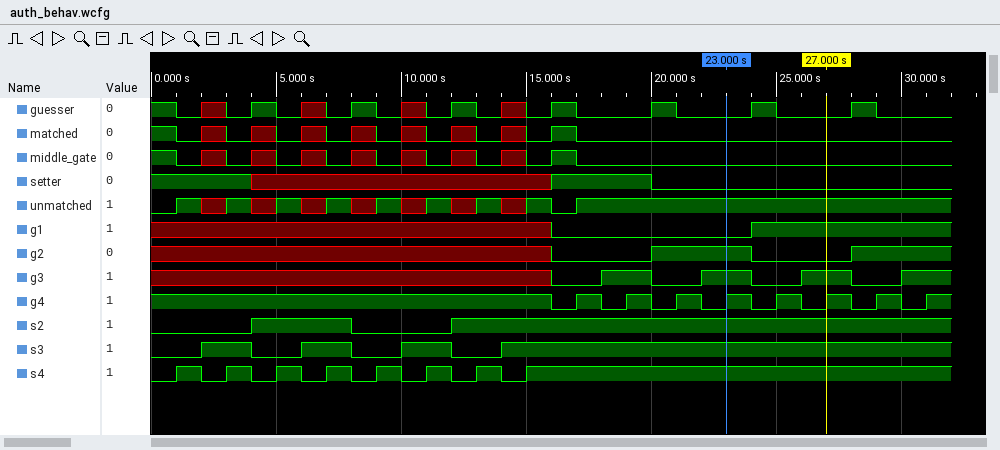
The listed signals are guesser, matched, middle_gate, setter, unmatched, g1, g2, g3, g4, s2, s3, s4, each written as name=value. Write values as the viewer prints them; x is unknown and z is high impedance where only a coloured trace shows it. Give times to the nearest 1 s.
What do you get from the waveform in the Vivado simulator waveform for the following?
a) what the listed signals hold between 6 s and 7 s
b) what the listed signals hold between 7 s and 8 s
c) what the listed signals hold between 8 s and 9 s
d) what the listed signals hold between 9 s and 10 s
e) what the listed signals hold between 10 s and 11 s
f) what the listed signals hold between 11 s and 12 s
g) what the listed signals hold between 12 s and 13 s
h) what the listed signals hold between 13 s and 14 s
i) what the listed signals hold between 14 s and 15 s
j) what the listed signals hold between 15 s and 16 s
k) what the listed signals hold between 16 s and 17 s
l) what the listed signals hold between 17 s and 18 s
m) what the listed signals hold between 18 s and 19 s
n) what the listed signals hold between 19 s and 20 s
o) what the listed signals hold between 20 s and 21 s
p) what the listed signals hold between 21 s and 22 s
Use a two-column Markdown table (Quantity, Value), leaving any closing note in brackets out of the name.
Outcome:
| Quantity | Value |
|---|---|
| what the listed signals hold between 6 s and 7 s | guesser=x, matched=x, middle_gate=x, setter=x, unmatched=x, g1=x, g2=x, g3=x, g4=1, s2=1, s3=1, s4=0 |
| what the listed signals hold between 7 s and 8 s | guesser=0, matched=0, middle_gate=0, setter=x, unmatched=1, g1=x, g2=x, g3=x, g4=1, s2=1, s3=1, s4=1 |
| what the listed signals hold between 8 s and 9 s | guesser=1, matched=x, middle_gate=x, setter=x, unmatched=x, g1=x, g2=x, g3=x, g4=1, s2=0, s3=0, s4=0 |
| what the listed signals hold between 9 s and 10 s | guesser=0, matched=0, middle_gate=0, setter=x, unmatched=1, g1=x, g2=x, g3=x, g4=1, s2=0, s3=0, s4=1 |
| what the listed signals hold between 10 s and 11 s | guesser=x, matched=x, middle_gate=x, setter=x, unmatched=x, g1=x, g2=x, g3=x, g4=1, s2=0, s3=1, s4=0 |
| what the listed signals hold between 11 s and 12 s | guesser=0, matched=0, middle_gate=0, setter=x, unmatched=1, g1=x, g2=x, g3=x, g4=1, s2=0, s3=1, s4=1 |
| what the listed signals hold between 12 s and 13 s | guesser=1, matched=x, middle_gate=x, setter=x, unmatched=x, g1=x, g2=x, g3=x, g4=1, s2=1, s3=0, s4=0 |
| what the listed signals hold between 13 s and 14 s | guesser=0, matched=0, middle_gate=0, setter=x, unmatched=1, g1=x, g2=x, g3=x, g4=1, s2=1, s3=0, s4=1 |
| what the listed signals hold between 14 s and 15 s | guesser=x, matched=x, middle_gate=x, setter=x, unmatched=x, g1=x, g2=x, g3=x, g4=1, s2=1, s3=1, s4=0 |
| what the listed signals hold between 15 s and 16 s | guesser=0, matched=0, middle_gate=0, setter=x, unmatched=1, g1=x, g2=x, g3=x, g4=1, s2=1, s3=1, s4=1 |
| what the listed signals hold between 16 s and 17 s | guesser=1, matched=1, middle_gate=1, setter=1, unmatched=0, g1=0, g2=0, g3=0, g4=0, s2=1, s3=1, s4=1 |
| what the listed signals hold between 17 s and 18 s | guesser=0, matched=0, middle_gate=0, setter=1, unmatched=1, g1=0, g2=0, g3=0, g4=1, s2=1, s3=1, s4=1 |
| what the listed signals hold between 18 s and 19 s | guesser=0, matched=0, middle_gate=0, setter=1, unmatched=1, g1=0, g2=0, g3=1, g4=0, s2=1, s3=1, s4=1 |
| what the listed signals hold between 19 s and 20 s | guesser=0, matched=0, middle_gate=0, setter=1, unmatched=1, g1=0, g2=0, g3=1, g4=1, s2=1, s3=1, s4=1 |
| what the listed signals hold between 20 s and 21 s | guesser=1, matched=0, middle_gate=0, setter=0, unmatched=1, g1=0, g2=1, g3=0, g4=0, s2=1, s3=1, s4=1 |
| what the listed signals hold between 21 s and 22 s | guesser=0, matched=0, middle_gate=0, setter=0, unmatched=1, g1=0, g2=1, g3=0, g4=1, s2=1, s3=1, s4=1 |
